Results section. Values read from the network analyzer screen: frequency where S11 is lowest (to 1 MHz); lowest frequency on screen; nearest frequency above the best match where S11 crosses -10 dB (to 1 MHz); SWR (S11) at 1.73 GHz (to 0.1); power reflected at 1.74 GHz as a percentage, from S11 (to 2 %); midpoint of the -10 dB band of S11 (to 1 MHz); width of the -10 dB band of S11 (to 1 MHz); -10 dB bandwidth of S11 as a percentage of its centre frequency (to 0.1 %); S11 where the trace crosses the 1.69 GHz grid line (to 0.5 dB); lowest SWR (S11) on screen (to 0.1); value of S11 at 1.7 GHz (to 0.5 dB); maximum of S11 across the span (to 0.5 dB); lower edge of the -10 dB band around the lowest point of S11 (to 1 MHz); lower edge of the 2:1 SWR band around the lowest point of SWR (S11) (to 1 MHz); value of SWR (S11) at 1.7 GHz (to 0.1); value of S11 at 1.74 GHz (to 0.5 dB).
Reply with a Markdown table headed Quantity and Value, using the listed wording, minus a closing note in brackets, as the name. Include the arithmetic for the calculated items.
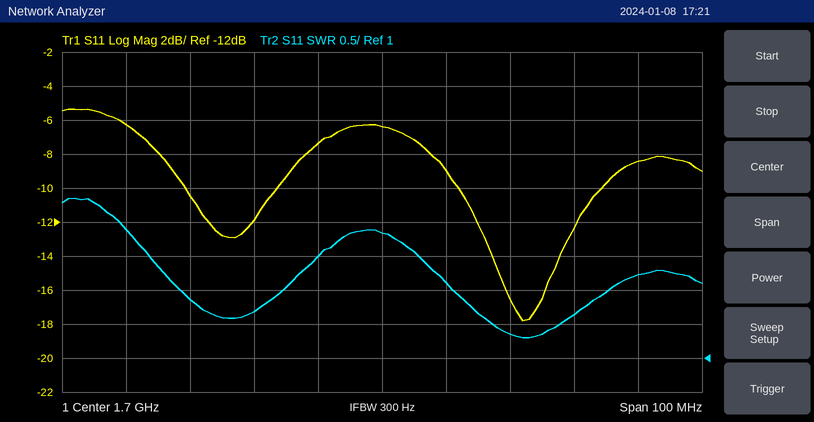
| Quantity | Value |
|---|---|
| frequency where S11 is lowest | 1.722 GHz |
| lowest frequency on screen | 1.65 GHz |
| nearest frequency above the best match where S11 crosses -10 dB | 1.734 GHz |
| SWR (S11) at 1.73 GHz | 1.6 |
| power reflected at 1.74 GHz as a percentage, from S11 | 10^(-8.5/10) ≈ 14 % |
| midpoint of the -10 dB band of S11 | 1.723 GHz |
| width of the -10 dB band of S11 | 1.734 GHz − 1.712 GHz = 22 MHz |
| -10 dB bandwidth of S11 as a percentage of its centre frequency | 22 MHz / 1.723 GHz ≈ 1.3 % |
| S11 where the trace crosses the 1.69 GHz grid line | -7.5 dB |
| lowest SWR (S11) on screen | 1.3 |
| value of S11 at 1.7 GHz | -6.5 dB |
| maximum of S11 across the span | -5.5 dB |
| lower edge of the -10 dB band around the lowest point of S11 | 1.712 GHz |
| lower edge of the 2:1 SWR band around the lowest point of SWR (S11) | 1.711 GHz |
| value of SWR (S11) at 1.7 GHz | 2.8 |
| value of S11 at 1.74 GHz | -8.5 dB |
